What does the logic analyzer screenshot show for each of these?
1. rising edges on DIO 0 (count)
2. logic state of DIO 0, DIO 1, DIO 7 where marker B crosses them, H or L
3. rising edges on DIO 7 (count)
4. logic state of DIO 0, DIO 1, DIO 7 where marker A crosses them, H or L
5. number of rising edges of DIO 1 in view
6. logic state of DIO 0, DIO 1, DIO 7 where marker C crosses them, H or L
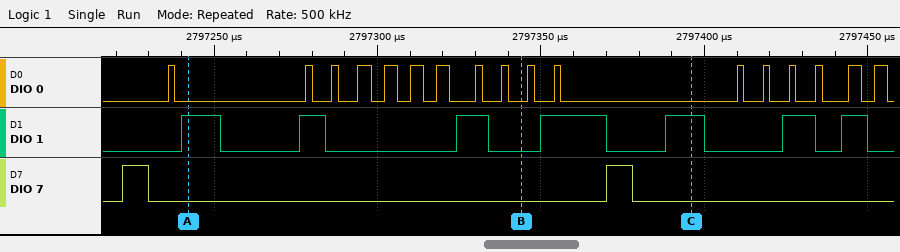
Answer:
17
DIO 0=L, DIO 1=L, DIO 7=L
2
DIO 0=L, DIO 1=H, DIO 7=L
7
DIO 0=L, DIO 1=H, DIO 7=L
